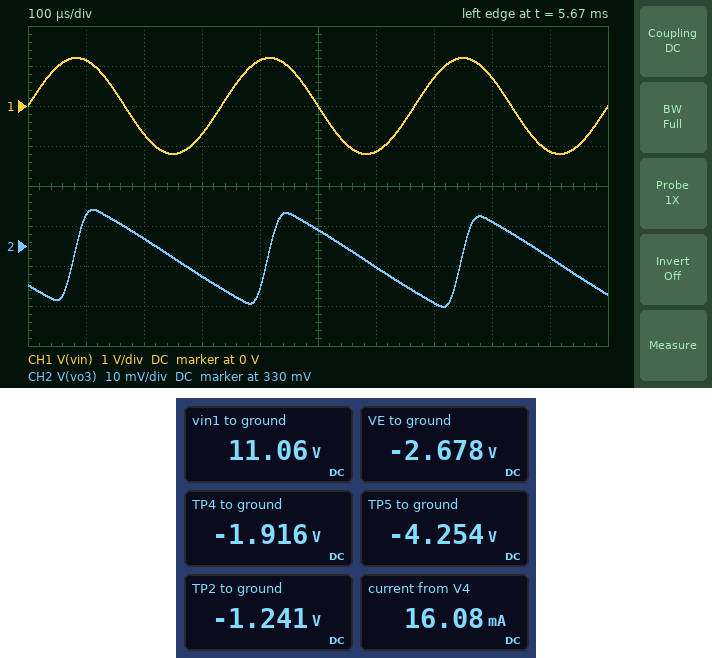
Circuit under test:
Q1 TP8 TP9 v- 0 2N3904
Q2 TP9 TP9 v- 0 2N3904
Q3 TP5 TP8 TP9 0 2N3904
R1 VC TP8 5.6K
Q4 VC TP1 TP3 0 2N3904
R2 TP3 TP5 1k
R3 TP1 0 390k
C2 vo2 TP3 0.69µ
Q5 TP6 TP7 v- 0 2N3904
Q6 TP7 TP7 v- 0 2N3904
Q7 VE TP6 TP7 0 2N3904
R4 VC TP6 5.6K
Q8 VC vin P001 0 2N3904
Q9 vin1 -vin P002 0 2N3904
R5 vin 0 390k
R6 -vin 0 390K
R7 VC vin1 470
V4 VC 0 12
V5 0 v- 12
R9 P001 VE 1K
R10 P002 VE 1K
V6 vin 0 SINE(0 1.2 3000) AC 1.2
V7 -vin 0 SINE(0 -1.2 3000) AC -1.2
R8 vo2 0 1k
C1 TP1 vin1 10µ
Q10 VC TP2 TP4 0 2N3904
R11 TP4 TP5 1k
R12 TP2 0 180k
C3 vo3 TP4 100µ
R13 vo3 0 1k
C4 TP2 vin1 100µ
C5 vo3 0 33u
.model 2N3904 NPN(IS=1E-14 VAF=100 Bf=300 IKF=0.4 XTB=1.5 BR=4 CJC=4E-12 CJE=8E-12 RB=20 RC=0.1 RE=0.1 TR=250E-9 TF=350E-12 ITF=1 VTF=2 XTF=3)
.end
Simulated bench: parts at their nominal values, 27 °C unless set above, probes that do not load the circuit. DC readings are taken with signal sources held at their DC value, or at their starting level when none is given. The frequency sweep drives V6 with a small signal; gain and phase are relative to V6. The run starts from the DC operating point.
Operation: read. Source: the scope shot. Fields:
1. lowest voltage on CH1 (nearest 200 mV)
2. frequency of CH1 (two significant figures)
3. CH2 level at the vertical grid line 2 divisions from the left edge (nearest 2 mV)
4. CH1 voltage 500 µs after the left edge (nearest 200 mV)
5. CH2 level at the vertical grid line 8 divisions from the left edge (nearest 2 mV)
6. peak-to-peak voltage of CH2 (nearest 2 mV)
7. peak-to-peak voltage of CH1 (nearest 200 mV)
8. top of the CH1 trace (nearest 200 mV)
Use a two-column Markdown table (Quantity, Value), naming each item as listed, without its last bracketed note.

| Quantity | Value |
|---|---|
| lowest voltage on CH1 | -1.2 V |
| frequency of CH1 | 3.0 kHz |
| CH2 level at the vertical grid line 2 divisions from the left edge | 332 mV |
| CH1 voltage 500 µs after the left edge | 0 V |
| CH2 level at the vertical grid line 8 divisions from the left edge | 336 mV |
| peak-to-peak voltage of CH2 | 24 mV |
| peak-to-peak voltage of CH1 | 2.4 V |
| top of the CH1 trace | 1.2 V |
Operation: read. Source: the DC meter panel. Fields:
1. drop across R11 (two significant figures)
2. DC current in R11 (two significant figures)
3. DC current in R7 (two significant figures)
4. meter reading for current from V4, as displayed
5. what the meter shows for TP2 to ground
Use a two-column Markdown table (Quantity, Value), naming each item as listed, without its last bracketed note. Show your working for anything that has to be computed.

| Quantity | Value |
|---|---|
| drop across R11 | -1.916 V - (-4.254 V) = 2.3 V |
| DC current in R11 | (-1.916 V - (-4.254 V)) / 1 kΩ = 2.3 mA |
| DC current in R7 | (12 V - 11.06 V) / 470 Ω = 2.0 mA |
| meter reading for current from V4, as displayed | 16.08 mA |
| what the meter shows for TP2 to ground | -1.241 V |
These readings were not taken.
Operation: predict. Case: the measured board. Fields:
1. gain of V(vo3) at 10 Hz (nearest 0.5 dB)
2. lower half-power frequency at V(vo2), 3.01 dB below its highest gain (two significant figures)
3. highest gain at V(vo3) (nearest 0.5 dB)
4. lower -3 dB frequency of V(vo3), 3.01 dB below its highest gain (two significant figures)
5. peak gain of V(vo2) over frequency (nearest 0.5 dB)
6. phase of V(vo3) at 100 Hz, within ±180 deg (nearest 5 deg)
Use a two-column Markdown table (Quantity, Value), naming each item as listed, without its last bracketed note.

| Quantity | Value |
|---|---|
| gain of V(vo3) at 10 Hz | -8.5 dB |
| lower half-power frequency at V(vo2), 3.01 dB below its highest gain | 190 Hz |
| highest gain at V(vo3) | -8.5 dB |
| lower -3 dB frequency of V(vo3), 3.01 dB below its highest gain | 1.2 Hz |
| peak gain of V(vo2) over frequency | -7.0 dB |
| phase of V(vo3) at 100 Hz, within ±180 deg | -10 deg |
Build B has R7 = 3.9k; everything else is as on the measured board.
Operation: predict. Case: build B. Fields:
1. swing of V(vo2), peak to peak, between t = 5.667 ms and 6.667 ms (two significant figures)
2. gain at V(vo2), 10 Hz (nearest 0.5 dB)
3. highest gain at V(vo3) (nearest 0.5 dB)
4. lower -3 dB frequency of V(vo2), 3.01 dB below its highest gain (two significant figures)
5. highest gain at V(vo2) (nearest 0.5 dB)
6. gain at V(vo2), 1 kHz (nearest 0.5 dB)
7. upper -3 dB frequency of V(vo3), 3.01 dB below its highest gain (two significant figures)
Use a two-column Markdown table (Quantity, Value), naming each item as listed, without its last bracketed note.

| Quantity | Value |
|---|---|
| swing of V(vo2), peak to peak, between t = 5.667 ms and 6.667 ms | 2.3 V |
| gain at V(vo2), 10 Hz | -15.0 dB |
| highest gain at V(vo3) | 9.5 dB |
| lower -3 dB frequency of V(vo2), 3.01 dB below its highest gain | 120 Hz |
| highest gain at V(vo2) | 8.0 dB |
| gain at V(vo2), 1 kHz | 6.5 dB |
| upper -3 dB frequency of V(vo3), 3.01 dB below its highest gain | 290 Hz |
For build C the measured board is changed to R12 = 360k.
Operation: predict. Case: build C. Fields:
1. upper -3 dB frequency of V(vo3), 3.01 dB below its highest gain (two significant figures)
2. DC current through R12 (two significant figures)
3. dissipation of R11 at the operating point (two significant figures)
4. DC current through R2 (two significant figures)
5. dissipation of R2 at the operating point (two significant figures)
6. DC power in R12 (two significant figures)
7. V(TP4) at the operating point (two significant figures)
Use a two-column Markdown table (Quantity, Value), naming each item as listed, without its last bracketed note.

| Quantity | Value |
|---|---|
| upper -3 dB frequency of V(vo3), 3.01 dB below its highest gain | 460 Hz |
| DC current through R12 | 6.0 µA |
| dissipation of R11 at the operating point | 4.2 mW |
| DC current through R2 | 2.0 mA |
| dissipation of R2 at the operating point | 3.9 mW |
| DC power in R12 | 13 µW |
| V(TP4) at the operating point | -2.8 V |
